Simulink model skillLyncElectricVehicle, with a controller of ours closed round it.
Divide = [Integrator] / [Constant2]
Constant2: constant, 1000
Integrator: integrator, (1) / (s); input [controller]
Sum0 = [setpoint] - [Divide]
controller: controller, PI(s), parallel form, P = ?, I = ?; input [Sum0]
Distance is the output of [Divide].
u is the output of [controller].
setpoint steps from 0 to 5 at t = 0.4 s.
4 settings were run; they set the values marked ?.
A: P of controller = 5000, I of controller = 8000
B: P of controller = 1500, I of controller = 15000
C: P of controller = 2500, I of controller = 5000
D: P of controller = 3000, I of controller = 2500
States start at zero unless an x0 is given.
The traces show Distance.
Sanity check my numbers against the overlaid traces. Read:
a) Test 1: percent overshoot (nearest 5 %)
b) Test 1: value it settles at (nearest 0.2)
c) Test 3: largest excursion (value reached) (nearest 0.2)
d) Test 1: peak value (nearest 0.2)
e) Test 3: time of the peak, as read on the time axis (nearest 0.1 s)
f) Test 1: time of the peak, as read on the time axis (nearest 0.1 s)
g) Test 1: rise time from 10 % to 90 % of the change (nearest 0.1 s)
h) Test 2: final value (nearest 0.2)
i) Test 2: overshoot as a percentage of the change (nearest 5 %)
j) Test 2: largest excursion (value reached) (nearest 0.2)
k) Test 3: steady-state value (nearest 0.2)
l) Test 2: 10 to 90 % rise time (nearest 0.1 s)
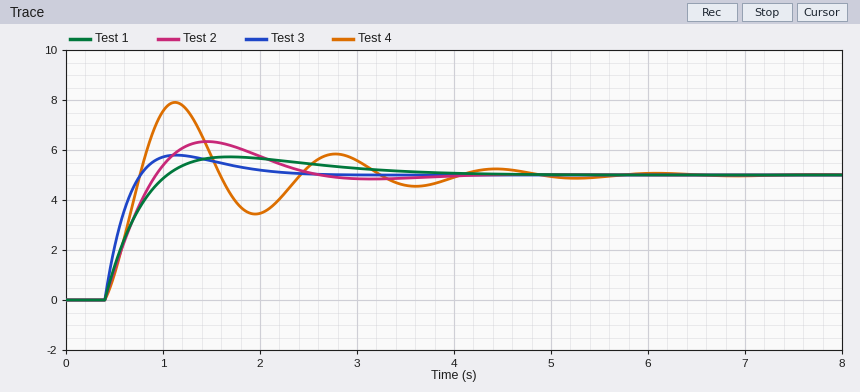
15 %
5.0
5.8
5.8
1.1 s
1.7 s
0.5 s
5.0
25 %
6.4
5.0
0.4 s
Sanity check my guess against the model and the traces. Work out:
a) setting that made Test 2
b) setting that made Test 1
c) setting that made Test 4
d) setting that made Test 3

C
D
B
A
